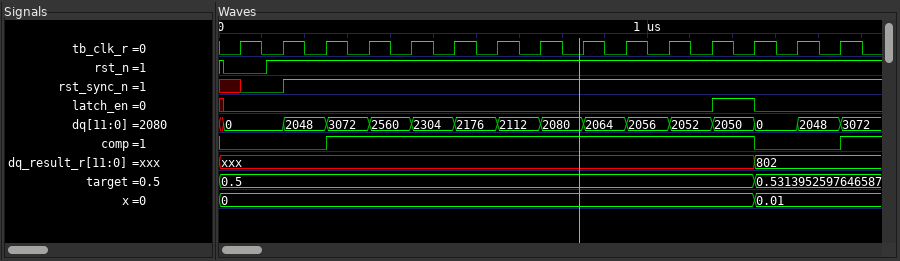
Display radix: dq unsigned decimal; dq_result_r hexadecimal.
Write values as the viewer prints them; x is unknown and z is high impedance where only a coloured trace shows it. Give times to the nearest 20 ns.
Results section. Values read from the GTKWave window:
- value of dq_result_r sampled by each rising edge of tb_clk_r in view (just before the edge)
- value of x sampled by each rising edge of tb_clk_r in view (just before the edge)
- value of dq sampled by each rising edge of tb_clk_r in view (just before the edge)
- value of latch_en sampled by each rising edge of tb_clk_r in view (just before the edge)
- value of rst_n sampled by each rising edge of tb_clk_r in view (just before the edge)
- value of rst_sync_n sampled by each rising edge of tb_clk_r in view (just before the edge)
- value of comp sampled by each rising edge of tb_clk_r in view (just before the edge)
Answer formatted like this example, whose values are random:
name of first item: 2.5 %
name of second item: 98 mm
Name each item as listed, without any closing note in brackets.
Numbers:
value of dq_result_r sampled by each rising edge of tb_clk_r in view: xxx, xxx, xxx, xxx, xxx, xxx, xxx, xxx, xxx, xxx, xxx, xxx, xxx, 802, 802
value of x sampled by each rising edge of tb_clk_r in view: 0, 0, 0, 0, 0, 0, 0, 0, 0, 0, 0, 0, 0, 0.01, 0.01
value of dq sampled by each rising edge of tb_clk_r in view: 0, 0, 2048, 3072, 2560, 2304, 2176, 2112, 2080, 2064, 2056, 2052, 2050, 0, 2048
value of latch_en sampled by each rising edge of tb_clk_r in view: 0 0 0 0 0 0 0 0 0 0 0 0 1 0 0
value of rst_n sampled by each rising edge of tb_clk_r in view: 0 1 1 1 1 1 1 1 1 1 1 1 1 1 1
value of rst_sync_n sampled by each rising edge of tb_clk_r in view: x 0 1 1 1 1 1 1 1 1 1 1 1 1 1
value of comp sampled by each rising edge of tb_clk_r in view: 0 0 0 1 1 1 1 1 1 1 1 1 1 0 0
